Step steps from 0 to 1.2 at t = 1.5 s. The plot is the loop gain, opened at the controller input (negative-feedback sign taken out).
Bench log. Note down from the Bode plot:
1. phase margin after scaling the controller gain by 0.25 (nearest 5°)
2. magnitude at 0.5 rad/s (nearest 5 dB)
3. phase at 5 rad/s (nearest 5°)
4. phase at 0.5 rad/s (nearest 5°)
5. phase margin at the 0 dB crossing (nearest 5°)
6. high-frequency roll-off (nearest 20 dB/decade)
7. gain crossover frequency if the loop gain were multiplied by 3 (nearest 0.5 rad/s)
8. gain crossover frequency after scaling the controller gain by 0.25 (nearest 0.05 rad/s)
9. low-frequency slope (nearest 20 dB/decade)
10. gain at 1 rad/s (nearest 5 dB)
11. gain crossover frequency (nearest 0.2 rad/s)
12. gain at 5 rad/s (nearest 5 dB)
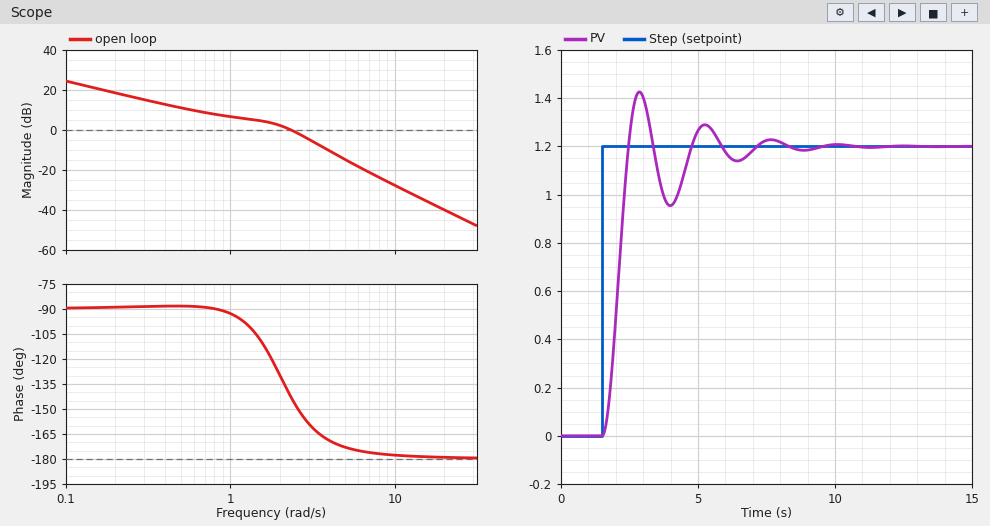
90°
10 dB
-175°
-90°
35°
-40 dB/decade
4.0 rad/s
0.45 rad/s
-20 dB/decade
5 dB
2.4 rad/s
-15 dB
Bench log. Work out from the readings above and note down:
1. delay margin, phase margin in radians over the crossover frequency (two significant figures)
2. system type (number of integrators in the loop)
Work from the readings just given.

0.25 s
1
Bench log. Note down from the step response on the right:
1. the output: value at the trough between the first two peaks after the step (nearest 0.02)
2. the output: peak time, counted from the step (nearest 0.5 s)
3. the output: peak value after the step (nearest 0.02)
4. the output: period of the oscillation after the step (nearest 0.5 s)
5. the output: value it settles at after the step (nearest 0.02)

0.96
1.5 s
1.42
2.5 s
1.20
